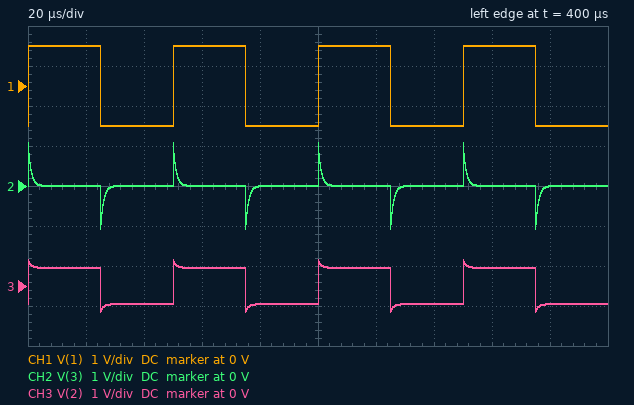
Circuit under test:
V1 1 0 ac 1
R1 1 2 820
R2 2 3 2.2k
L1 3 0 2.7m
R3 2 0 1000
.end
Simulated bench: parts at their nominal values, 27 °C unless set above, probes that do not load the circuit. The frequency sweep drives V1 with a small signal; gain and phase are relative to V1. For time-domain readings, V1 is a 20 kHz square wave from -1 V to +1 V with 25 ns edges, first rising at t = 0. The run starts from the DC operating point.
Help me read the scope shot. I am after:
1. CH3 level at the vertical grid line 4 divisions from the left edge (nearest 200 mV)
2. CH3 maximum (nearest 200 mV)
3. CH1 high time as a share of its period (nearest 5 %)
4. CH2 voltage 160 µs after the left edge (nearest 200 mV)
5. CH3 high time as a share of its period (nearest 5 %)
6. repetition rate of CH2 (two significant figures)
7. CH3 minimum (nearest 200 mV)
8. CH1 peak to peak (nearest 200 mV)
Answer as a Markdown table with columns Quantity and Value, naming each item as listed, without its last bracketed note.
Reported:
| Quantity | Value |
|---|---|
| CH3 level at the vertical grid line 4 divisions from the left edge | -400 mV |
| CH3 maximum | 600 mV |
| CH1 high time as a share of its period | 50 % |
| CH2 voltage 160 µs after the left edge | 0 V |
| CH3 high time as a share of its period | 50 % |
| repetition rate of CH2 | 20 kHz |
| CH3 minimum | -600 mV |
| CH1 peak to peak | 2.0 V |
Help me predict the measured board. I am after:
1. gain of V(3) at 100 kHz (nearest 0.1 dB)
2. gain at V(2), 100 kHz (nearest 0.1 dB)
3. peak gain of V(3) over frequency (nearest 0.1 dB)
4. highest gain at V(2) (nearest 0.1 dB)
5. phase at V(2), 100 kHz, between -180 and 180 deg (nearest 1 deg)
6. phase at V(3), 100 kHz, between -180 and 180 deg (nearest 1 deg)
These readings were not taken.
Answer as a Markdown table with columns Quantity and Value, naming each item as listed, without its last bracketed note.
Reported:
| Quantity | Value |
|---|---|
| gain of V(3) at 100 kHz | -10.6 dB |
| gain at V(2), 100 kHz | -6.3 dB |
| peak gain of V(3) over frequency | -5.2 dB |
| highest gain at V(2) | -5.2 dB |
| phase at V(2), 100 kHz, between -180 and 180 deg | 5 deg |
| phase at V(3), 100 kHz, between -180 and 180 deg | 57 deg |
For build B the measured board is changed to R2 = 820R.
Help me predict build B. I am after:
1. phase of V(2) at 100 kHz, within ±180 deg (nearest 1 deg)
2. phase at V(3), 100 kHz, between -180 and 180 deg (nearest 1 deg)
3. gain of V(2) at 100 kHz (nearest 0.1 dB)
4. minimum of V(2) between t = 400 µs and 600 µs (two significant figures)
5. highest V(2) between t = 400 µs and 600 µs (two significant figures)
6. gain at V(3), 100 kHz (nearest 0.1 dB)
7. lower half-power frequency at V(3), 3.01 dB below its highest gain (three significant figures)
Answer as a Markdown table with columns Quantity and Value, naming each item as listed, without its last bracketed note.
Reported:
| Quantity | Value |
|---|---|
| phase of V(2) at 100 kHz, within ±180 deg | 11 deg |
| phase at V(3), 100 kHz, between -180 and 180 deg | 37 deg |
| gain of V(2) at 100 kHz | -6.2 dB |
| minimum of V(2) between t = 400 µs and 600 µs | -740 mV |
| highest V(2) between t = 400 µs and 600 µs | 740 mV |
| gain at V(3), 100 kHz | -7.1 dB |
| lower half-power frequency at V(3), 3.01 dB below its highest gain | 74.9 kHz |
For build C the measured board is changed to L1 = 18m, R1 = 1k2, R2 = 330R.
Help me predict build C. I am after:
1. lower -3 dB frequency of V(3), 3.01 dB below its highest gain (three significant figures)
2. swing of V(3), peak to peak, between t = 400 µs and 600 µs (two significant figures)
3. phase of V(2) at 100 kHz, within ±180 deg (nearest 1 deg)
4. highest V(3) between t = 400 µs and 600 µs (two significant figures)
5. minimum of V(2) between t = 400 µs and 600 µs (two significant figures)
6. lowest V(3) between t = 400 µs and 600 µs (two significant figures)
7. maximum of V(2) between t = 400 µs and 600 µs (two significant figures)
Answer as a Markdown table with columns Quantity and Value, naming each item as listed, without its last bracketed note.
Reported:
| Quantity | Value |
|---|---|
| lower -3 dB frequency of V(3), 3.01 dB below its highest gain | 7.74 kHz |
| swing of V(3), peak to peak, between t = 400 µs and 600 µs | 1.4 V |
| phase of V(2) at 100 kHz, within ±180 deg | 3 deg |
| highest V(3) between t = 400 µs and 600 µs | 700 mV |
| minimum of V(2) between t = 400 µs and 600 µs | -610 mV |
| lowest V(3) between t = 400 µs and 600 µs | -700 mV |
| maximum of V(2) between t = 400 µs and 600 µs | 610 mV |
